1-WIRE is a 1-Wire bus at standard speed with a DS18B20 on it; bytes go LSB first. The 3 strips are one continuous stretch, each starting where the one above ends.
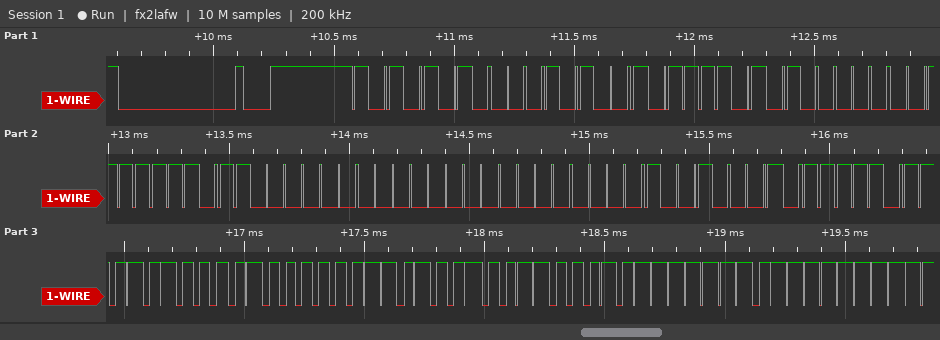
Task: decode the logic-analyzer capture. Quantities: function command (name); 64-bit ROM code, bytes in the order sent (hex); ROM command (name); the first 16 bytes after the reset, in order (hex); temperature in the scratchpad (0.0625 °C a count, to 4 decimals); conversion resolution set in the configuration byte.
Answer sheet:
Read Scratchpad
28 BD 02 7E 03 00 00 89
Match ROM
55 28 BD 02 7E 03 00 00 89 BE 15 02 4B 46 7F FF
33.3125 °C
12 bits
